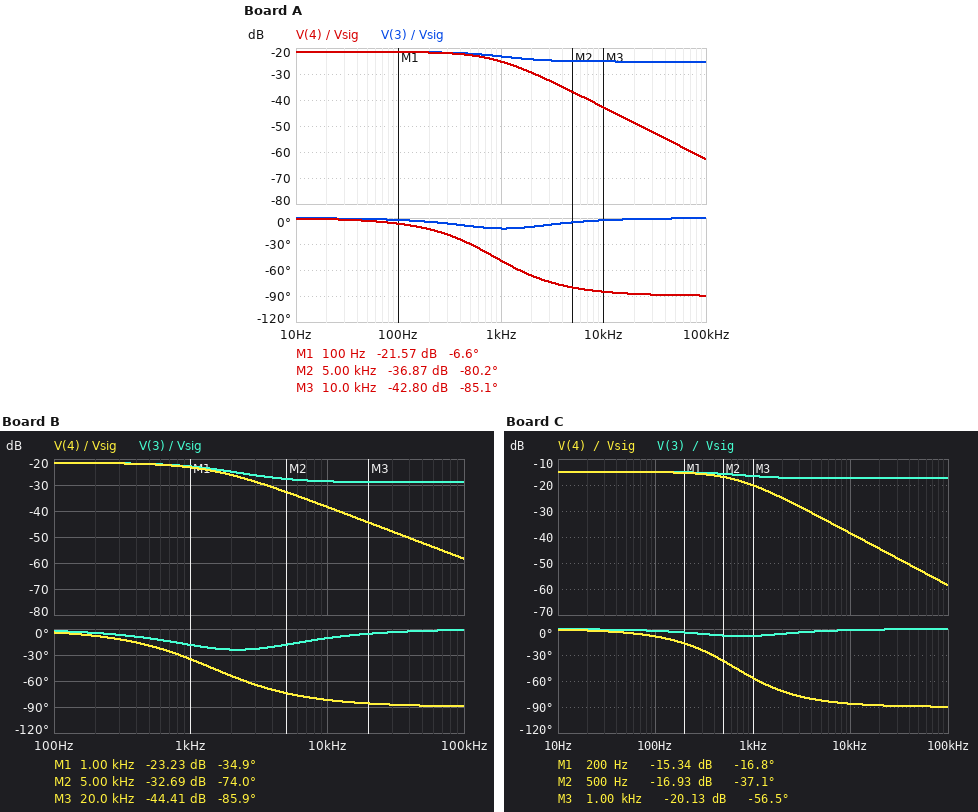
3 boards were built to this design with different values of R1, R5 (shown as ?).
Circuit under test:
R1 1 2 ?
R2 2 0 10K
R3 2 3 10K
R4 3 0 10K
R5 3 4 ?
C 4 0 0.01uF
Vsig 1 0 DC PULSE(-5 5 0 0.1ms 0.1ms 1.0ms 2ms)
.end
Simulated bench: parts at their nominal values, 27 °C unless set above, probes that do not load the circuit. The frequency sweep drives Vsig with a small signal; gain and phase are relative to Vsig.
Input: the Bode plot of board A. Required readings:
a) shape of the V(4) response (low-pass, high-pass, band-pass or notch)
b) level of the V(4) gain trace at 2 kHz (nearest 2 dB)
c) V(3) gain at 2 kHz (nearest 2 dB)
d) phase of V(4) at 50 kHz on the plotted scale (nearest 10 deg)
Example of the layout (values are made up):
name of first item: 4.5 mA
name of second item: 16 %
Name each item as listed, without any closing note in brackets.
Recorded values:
shape of the V(4) response: low-pass
level of the V(4) gain trace at 2 kHz: -30 dB
V(3) gain at 2 kHz: -24 dB
phase of V(4) at 50 kHz on the plotted scale: -90 deg
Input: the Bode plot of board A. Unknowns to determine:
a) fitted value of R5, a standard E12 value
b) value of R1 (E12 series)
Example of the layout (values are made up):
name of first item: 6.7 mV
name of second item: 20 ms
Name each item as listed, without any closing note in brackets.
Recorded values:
fitted value of R5, a standard E12 value: 12 kΩ
value of R1: 33 kΩ
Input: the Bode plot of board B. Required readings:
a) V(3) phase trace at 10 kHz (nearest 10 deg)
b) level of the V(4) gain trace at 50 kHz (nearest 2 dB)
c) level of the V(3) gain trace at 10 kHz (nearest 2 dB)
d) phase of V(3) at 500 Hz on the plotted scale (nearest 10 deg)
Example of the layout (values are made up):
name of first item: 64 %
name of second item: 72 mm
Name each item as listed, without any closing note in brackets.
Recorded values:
V(3) phase trace at 10 kHz: -10 deg
level of the V(4) gain trace at 50 kHz: -52 dB
level of the V(3) gain trace at 10 kHz: -28 dB
phase of V(3) at 500 Hz on the plotted scale: -10 deg
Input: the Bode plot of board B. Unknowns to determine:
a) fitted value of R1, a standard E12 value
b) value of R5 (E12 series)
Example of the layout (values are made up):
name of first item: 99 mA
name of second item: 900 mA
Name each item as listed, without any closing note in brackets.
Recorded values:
fitted value of R1, a standard E12 value: 33 kΩ
value of R5: 4.7 kΩ
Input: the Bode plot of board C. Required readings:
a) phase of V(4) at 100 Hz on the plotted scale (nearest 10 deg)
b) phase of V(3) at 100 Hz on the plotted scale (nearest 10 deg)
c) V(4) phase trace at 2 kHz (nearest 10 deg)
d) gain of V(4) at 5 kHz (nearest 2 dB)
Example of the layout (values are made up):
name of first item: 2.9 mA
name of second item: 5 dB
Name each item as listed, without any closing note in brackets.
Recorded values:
phase of V(4) at 100 Hz on the plotted scale: -10 deg
phase of V(3) at 100 Hz on the plotted scale: 0 deg
V(4) phase trace at 2 kHz: -70 deg
gain of V(4) at 5 kHz: -32 dB
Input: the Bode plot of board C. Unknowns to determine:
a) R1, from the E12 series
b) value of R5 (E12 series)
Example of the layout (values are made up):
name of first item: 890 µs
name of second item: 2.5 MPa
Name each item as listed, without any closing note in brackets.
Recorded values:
R1, from the E12 series: 12 kΩ
value of R5: 18 kΩ
